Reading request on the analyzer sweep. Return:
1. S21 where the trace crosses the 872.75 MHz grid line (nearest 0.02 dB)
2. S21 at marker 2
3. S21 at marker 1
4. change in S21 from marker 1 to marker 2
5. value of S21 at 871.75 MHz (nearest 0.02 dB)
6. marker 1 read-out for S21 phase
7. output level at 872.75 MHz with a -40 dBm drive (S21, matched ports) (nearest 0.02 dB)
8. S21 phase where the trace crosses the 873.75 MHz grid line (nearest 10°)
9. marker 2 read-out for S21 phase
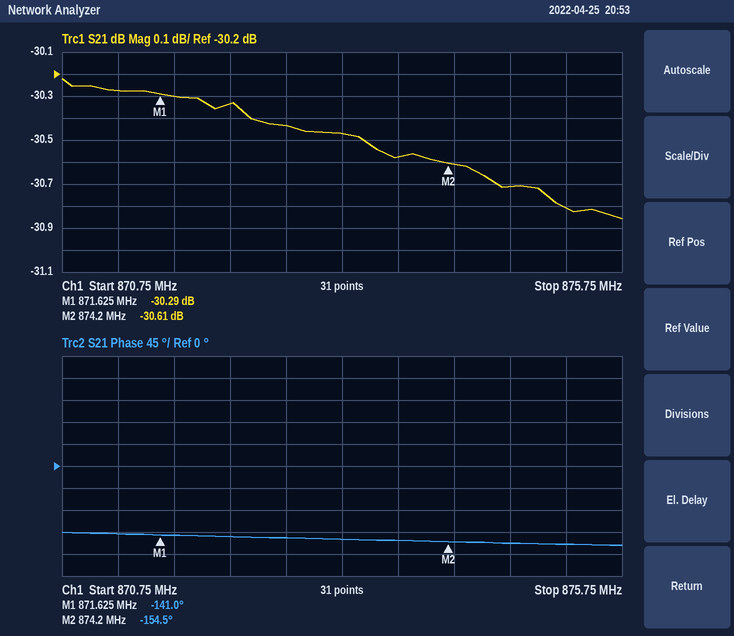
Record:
-30.44 dB
-30.61 dB
-30.29 dB
-0.32 dB
-30.30 dB
-141.0°
-70.44 dBm
-150°
-154.5°
